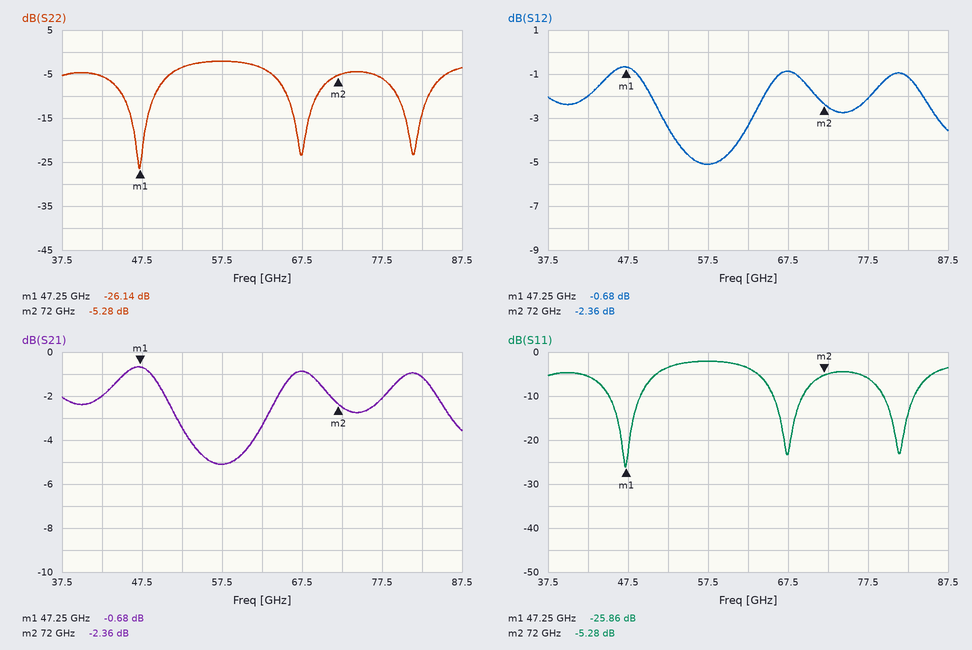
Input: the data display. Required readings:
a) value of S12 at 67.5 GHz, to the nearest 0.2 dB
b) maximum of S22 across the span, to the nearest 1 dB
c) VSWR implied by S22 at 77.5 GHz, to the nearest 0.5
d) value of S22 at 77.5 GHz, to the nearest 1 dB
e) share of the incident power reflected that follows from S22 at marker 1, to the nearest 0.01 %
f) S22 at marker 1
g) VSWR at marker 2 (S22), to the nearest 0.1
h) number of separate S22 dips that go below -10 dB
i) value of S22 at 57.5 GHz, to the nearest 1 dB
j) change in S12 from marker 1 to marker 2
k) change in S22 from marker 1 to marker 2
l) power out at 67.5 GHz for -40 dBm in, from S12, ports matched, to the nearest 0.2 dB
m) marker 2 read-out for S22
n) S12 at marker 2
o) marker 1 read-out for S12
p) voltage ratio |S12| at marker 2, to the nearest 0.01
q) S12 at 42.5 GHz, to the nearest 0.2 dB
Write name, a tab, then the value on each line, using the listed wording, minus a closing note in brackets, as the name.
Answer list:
value of S12 at 67.5 GHz, to the nearest 0.2 dB	-0.8 dB
maximum of S22 across the span, to the nearest 1 dB	-2 dB
VSWR implied by S22 at 77.5 GHz, to the nearest 0.5	3.0
value of S22 at 77.5 GHz, to the nearest 1 dB	-6 dB
share of the incident power reflected that follows from S22 at marker 1, to the nearest 0.01 %	0.24 %
S22 at marker 1	-26.14 dB
VSWR at marker 2 (S22), to the nearest 0.1	3.4
number of separate S22 dips that go below -10 dB	3
value of S22 at 57.5 GHz, to the nearest 1 dB	-2 dB
change in S12 from marker 1 to marker 2	-1.68 dB
change in S22 from marker 1 to marker 2	20.86 dB
power out at 67.5 GHz for -40 dBm in, from S12, ports matched, to the nearest 0.2 dB	-40.8 dBm
marker 2 read-out for S22	-5.28 dB
S12 at marker 2	-2.36 dB
marker 1 read-out for S12	-0.68 dB
voltage ratio |S12| at marker 2, to the nearest 0.01	0.76
S12 at 42.5 GHz, to the nearest 0.2 dB	-2.0 dB
